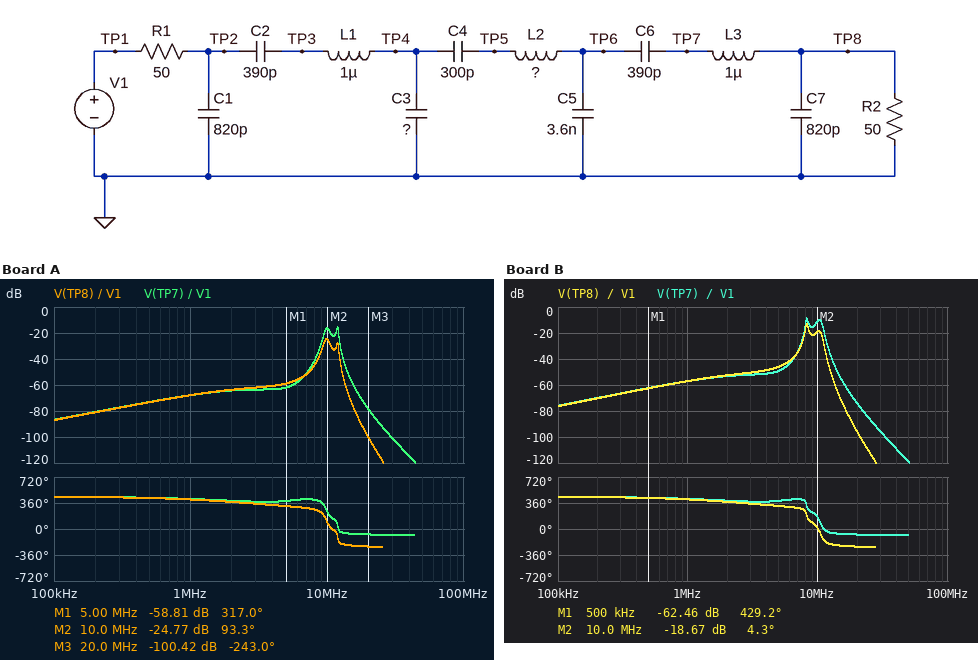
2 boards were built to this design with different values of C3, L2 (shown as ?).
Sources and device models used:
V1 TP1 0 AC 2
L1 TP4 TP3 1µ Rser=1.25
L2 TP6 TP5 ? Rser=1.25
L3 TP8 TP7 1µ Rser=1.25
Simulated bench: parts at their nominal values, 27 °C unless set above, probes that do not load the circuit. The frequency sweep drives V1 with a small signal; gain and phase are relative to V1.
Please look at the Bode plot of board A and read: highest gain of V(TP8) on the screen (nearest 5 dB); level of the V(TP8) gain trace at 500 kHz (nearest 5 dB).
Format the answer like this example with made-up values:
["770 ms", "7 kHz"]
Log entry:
["-25 dB", "-75 dB"]
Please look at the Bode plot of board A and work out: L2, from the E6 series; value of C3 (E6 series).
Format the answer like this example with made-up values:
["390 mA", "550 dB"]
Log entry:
["680 nH", "6.8 nF"]
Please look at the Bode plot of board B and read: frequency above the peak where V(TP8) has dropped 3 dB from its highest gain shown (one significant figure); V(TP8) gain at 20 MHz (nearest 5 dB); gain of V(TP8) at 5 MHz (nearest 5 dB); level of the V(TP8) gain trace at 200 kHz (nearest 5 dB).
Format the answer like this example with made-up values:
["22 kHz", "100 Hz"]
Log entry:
["8 MHz", "-95 dB", "-45 dB", "-70 dB"]
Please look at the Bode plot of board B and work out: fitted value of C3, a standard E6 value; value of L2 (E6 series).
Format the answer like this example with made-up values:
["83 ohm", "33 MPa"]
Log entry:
["1.5 nF", "1.5 µH"]
